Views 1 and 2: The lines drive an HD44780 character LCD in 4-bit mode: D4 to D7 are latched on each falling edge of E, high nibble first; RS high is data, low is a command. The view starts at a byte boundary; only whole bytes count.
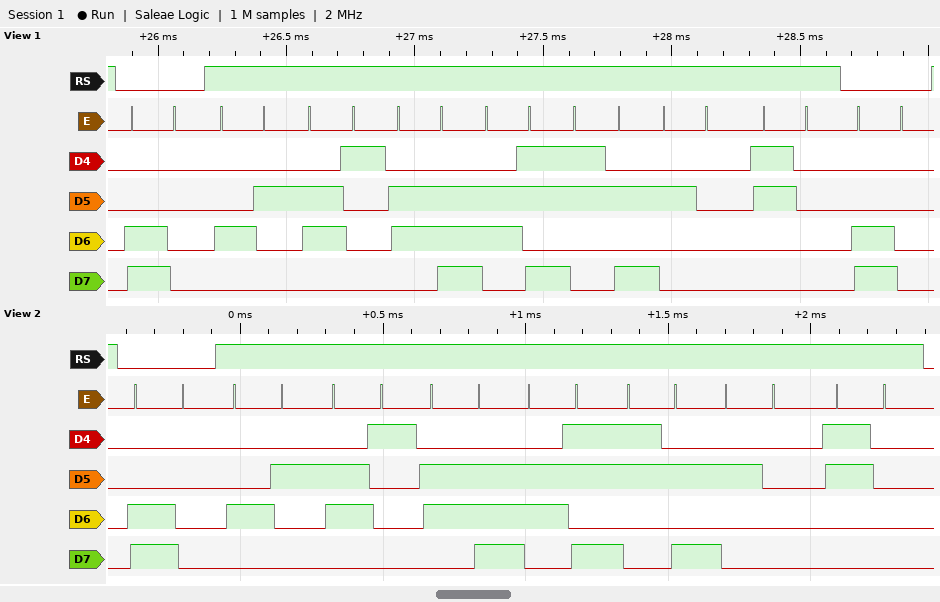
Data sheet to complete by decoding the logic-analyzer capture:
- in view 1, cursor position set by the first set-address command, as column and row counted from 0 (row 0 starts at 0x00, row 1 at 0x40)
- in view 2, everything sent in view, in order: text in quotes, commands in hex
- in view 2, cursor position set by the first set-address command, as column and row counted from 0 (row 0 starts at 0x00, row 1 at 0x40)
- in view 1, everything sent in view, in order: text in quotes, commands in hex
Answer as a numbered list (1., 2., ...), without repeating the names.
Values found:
1. column 0, row 1
2. 0xC0 "Bank: 0"
3. column 0, row 1
4. 0xC0 "Bank: 0" 0xC0
